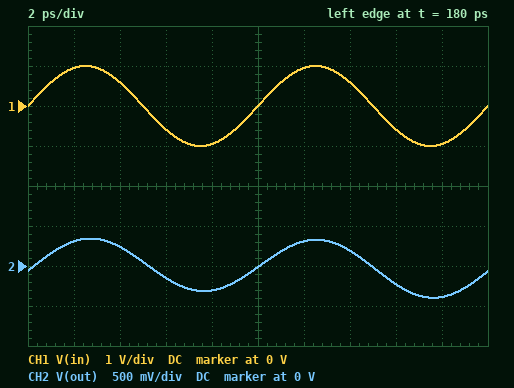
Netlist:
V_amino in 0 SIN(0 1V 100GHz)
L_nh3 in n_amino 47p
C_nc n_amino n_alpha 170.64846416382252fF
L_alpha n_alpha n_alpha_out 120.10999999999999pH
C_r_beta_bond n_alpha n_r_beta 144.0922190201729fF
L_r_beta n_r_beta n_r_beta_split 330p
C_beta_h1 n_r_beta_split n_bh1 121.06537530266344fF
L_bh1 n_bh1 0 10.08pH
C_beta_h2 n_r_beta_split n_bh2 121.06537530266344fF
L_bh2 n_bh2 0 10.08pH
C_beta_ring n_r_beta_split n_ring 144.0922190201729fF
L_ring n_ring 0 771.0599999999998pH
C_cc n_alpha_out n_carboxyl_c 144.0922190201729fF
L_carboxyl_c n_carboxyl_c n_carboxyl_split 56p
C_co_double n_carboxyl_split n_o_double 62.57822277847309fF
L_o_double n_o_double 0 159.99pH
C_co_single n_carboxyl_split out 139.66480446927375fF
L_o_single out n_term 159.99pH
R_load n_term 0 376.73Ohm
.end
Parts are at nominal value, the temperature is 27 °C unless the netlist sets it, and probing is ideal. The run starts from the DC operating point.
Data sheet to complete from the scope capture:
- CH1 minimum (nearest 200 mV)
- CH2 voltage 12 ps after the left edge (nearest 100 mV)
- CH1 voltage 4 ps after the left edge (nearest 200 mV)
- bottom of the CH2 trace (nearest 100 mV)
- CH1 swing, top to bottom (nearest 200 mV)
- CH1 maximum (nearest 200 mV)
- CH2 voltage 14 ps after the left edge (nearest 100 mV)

-1.0 V
300 mV
600 mV
-400 mV
2.0 V
1.0 V
200 mV
